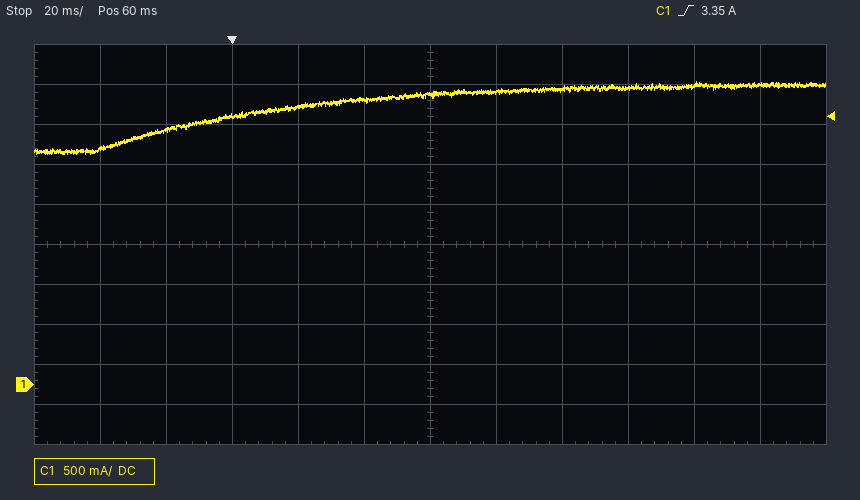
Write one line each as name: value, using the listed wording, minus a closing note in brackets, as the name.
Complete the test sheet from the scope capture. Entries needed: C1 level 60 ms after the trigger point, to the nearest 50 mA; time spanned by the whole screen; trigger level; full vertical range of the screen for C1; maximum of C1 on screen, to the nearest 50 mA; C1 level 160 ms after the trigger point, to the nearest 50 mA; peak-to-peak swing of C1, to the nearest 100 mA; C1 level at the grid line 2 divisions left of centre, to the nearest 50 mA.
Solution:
C1 level 60 ms after the trigger point, to the nearest 50 mA: 3.60 A
time spanned by the whole screen: 240 ms
trigger level: 3.35 A
full vertical range of the screen for C1: 5 A
maximum of C1 on screen, to the nearest 50 mA: 3.80 A
C1 level 160 ms after the trigger point, to the nearest 50 mA: 3.75 A
peak-to-peak swing of C1, to the nearest 100 mA: 900 mA
C1 level at the grid line 2 divisions left of centre, to the nearest 50 mA: 3.45 A
